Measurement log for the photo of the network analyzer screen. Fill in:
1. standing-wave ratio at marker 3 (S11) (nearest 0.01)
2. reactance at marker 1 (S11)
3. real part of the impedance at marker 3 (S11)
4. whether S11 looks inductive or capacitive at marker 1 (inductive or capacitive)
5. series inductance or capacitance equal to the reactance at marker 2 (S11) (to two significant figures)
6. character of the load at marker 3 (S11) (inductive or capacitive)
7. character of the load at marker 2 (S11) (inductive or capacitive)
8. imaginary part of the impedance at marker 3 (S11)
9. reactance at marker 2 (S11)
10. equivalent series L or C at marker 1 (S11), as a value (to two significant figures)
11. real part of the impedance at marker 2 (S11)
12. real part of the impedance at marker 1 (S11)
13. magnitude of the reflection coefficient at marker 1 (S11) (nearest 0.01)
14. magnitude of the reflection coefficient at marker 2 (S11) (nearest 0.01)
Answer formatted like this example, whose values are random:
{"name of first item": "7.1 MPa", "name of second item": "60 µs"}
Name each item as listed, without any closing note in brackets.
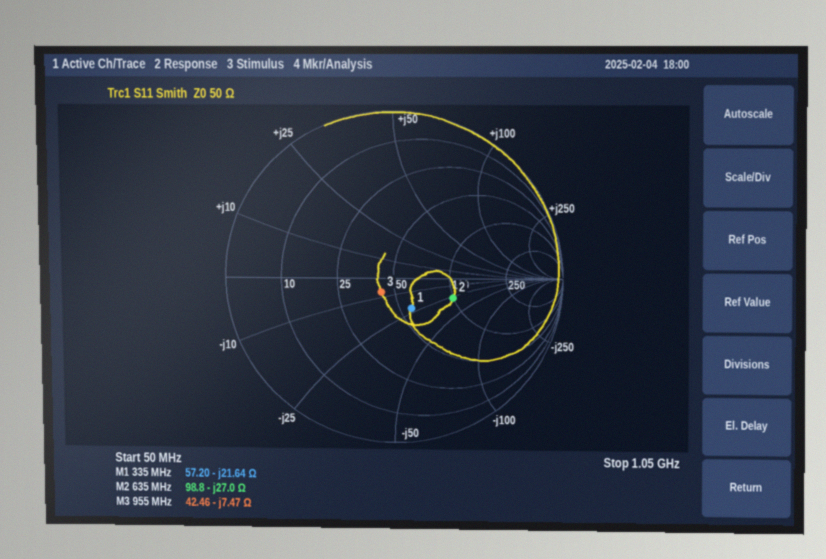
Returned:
{"standing-wave ratio at marker 3 (S11)": "1.26", "reactance at marker 1": "-21.64 Ω", "real part of the impedance at marker 3": "42.46 Ω", "whether S11 looks inductive or capacitive at marker 1": "capacitive", "series inductance or capacitance equal to the reactance at marker 2 (S11)": "9.3 pF", "character of the load at marker 3 (S11)": "capacitive", "character of the load at marker 2 (S11)": "capacitive", "imaginary part of the impedance at marker 3": "-7.47 Ω", "reactance at marker 2": "-27.0 Ω", "equivalent series L or C at marker 1 (S11), as a value": "22 pF", "real part of the impedance at marker 2": "98.8 Ω", "real part of the impedance at marker 1": "57.20 Ω", "magnitude of the reflection coefficient at marker 1 (S11)": "0.21", "magnitude of the reflection coefficient at marker 2 (S11)": "0.37"}
